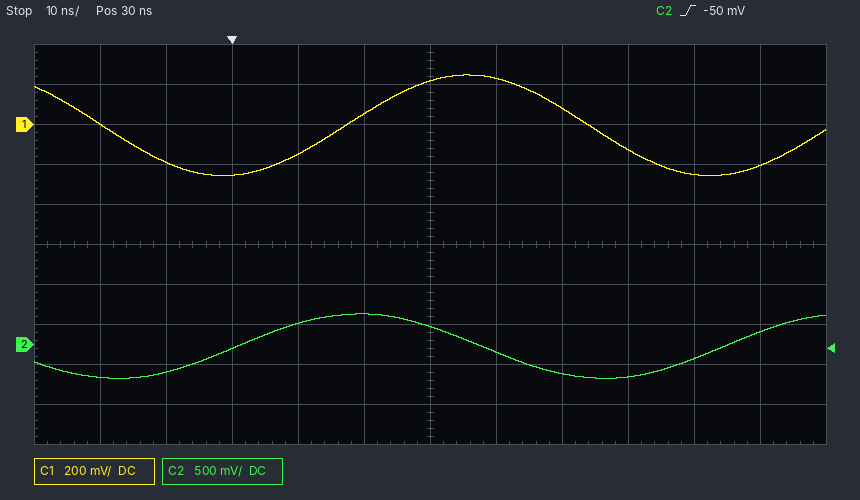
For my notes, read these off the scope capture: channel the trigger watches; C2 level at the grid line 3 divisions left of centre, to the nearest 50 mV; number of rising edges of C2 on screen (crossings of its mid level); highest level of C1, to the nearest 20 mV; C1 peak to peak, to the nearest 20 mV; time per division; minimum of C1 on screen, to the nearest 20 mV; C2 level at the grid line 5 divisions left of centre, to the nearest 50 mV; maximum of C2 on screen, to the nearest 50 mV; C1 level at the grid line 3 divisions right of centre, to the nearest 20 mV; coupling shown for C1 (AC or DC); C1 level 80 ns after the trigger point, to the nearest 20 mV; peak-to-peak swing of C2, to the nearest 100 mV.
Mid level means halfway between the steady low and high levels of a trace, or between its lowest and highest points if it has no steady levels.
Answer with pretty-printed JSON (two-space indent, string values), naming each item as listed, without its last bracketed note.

{
  "channel the trigger watches": "C2",
  "C2 level at the grid line 3 divisions left of centre, to the nearest 50 mV": "-50 mV",
  "number of rising edges of C2 on screen": "2",
  "highest level of C1, to the nearest 20 mV": "240 mV",
  "C1 peak to peak, to the nearest 20 mV": "500 mV",
  "time per division": "10 ns",
  "minimum of C1 on screen, to the nearest 20 mV": "-260 mV",
  "C2 level at the grid line 5 divisions left of centre, to the nearest 50 mV": "-400 mV",
  "maximum of C2 on screen, to the nearest 50 mV": "400 mV",
  "C1 level at the grid line 3 divisions right of centre, to the nearest 20 mV": "-120 mV",
  "coupling shown for C1": "DC",
  "C1 level 80 ns after the trigger point, to the nearest 20 mV": "-200 mV",
  "peak-to-peak swing of C2, to the nearest 100 mV": "800 mV"
}
